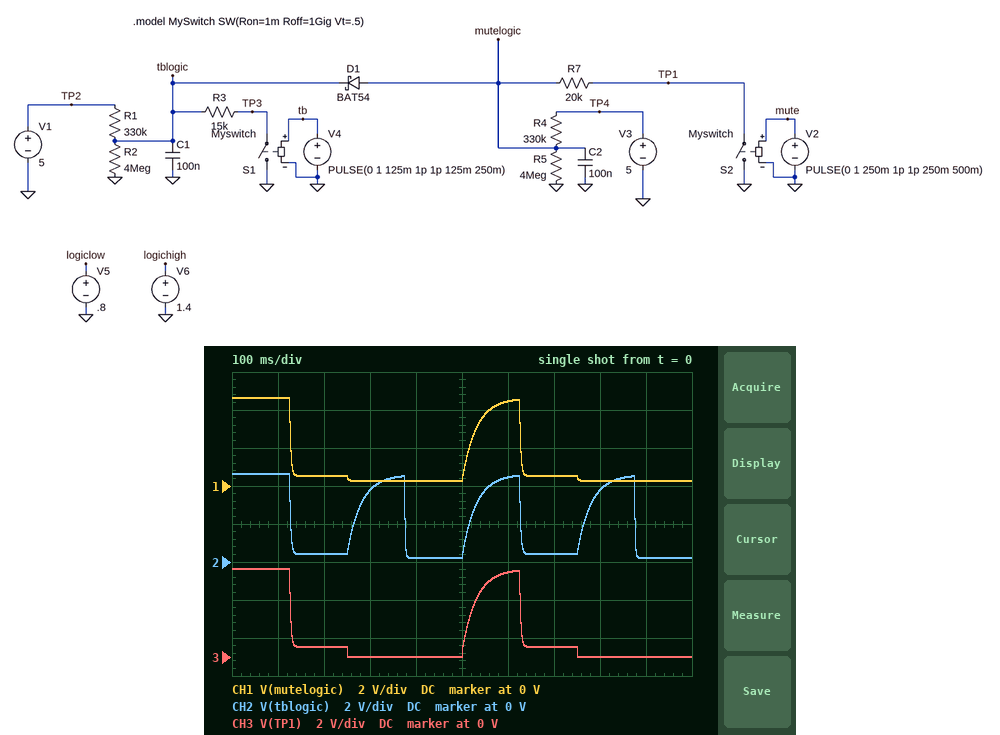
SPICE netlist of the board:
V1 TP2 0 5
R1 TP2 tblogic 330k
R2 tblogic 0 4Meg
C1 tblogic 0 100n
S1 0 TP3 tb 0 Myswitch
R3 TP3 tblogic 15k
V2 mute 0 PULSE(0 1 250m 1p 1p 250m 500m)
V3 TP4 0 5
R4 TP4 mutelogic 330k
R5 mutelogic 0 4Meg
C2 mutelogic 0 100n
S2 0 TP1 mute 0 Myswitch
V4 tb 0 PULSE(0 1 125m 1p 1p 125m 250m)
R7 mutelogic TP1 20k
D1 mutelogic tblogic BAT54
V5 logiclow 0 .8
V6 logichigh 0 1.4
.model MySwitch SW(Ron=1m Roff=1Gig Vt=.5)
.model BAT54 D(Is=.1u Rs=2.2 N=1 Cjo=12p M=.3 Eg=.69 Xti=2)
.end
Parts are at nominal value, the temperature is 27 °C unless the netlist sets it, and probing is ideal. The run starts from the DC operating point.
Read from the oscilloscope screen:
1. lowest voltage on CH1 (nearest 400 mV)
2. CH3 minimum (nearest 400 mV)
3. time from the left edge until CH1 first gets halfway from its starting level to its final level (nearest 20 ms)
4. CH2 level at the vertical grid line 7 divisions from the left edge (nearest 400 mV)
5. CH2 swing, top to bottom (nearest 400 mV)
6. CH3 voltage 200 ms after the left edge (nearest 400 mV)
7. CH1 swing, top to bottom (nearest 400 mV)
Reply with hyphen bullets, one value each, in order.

- 400 mV
- 0 V
- 120 ms
- 400 mV
- 4.4 V
- 400 mV
- 4.4 V
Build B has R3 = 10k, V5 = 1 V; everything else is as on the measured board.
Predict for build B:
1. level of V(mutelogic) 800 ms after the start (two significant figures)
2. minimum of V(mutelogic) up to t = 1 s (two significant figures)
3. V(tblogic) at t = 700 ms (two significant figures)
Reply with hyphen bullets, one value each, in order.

- 290 mV
- 250 mV
- 280 mV
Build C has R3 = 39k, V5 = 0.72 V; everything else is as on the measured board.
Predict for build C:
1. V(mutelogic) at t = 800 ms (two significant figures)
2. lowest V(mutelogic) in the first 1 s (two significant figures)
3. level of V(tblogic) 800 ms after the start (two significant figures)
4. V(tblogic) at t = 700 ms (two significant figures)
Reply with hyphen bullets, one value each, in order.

- 290 mV
- 290 mV
- 3.9 V
- 930 mV
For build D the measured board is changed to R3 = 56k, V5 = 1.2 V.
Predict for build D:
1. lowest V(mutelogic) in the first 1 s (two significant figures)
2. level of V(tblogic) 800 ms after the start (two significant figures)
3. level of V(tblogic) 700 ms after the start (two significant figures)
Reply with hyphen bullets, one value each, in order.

- 290 mV
- 3.9 V
- 1.2 V
